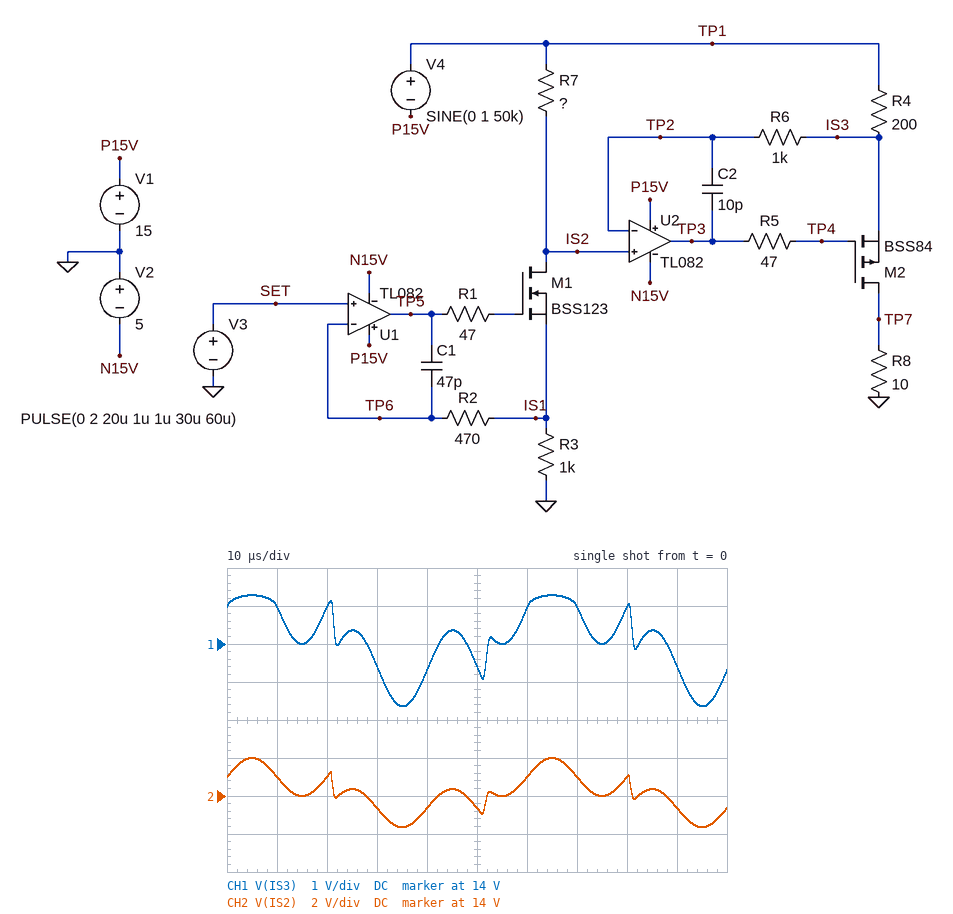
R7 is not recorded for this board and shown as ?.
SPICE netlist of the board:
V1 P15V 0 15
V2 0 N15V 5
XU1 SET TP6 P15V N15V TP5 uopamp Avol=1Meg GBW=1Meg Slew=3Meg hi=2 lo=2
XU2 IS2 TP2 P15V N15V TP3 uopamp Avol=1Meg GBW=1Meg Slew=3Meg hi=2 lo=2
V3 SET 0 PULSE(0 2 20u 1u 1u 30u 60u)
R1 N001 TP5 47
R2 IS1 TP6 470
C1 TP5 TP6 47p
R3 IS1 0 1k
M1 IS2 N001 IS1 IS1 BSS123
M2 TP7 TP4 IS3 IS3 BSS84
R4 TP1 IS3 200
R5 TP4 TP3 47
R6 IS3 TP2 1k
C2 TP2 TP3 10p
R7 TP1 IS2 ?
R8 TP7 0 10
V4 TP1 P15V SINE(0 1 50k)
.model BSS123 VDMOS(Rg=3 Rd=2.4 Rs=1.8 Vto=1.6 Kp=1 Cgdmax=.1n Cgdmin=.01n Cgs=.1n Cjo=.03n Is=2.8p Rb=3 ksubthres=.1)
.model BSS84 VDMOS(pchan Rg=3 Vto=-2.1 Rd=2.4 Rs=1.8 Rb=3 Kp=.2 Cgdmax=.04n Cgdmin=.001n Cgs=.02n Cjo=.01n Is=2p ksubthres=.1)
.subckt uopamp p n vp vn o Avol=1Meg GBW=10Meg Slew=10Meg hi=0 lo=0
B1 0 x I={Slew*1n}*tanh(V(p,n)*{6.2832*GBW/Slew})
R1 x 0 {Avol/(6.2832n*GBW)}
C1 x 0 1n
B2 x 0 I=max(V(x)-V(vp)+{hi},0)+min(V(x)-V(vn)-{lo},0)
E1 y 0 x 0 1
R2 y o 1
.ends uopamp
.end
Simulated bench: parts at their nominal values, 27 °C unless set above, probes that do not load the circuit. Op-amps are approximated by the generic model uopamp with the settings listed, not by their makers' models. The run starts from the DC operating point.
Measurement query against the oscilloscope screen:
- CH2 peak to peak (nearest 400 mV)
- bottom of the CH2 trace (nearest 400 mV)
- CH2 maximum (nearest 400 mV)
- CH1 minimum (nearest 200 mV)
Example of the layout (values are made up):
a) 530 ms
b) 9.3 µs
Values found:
a) 3.6 V
b) 12.4 V
c) 16.0 V
d) 12.4 V
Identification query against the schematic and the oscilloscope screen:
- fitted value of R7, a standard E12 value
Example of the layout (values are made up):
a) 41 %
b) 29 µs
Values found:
a) 820 Ω
